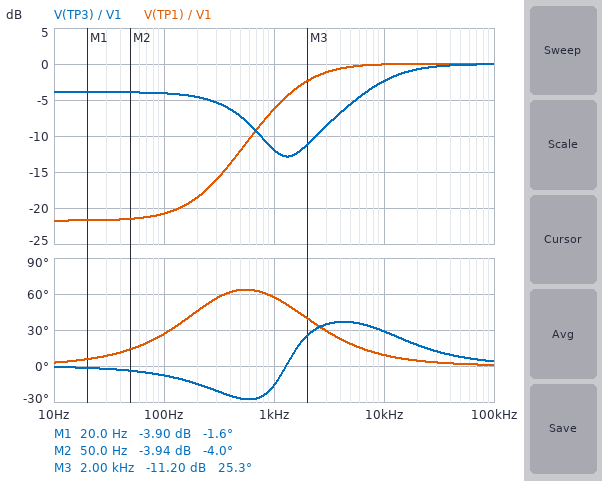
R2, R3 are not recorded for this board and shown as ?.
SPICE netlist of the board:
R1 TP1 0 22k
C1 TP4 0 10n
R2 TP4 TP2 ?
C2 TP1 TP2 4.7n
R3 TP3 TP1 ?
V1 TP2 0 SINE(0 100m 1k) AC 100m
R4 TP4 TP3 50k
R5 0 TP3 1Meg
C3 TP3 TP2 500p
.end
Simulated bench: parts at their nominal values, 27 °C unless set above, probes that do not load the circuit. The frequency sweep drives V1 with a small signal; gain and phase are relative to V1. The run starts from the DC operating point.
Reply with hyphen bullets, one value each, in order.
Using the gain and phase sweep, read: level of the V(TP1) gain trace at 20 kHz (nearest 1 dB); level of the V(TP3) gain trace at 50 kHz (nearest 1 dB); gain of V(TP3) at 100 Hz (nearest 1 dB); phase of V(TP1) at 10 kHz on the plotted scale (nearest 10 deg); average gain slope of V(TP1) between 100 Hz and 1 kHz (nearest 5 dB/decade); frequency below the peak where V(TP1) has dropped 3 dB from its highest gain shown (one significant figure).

- 0 dB
- 0 dB
- -4 dB
- 10 deg
- 15 dB/decade
- 2 kHz
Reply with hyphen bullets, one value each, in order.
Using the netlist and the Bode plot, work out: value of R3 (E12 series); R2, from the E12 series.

- 150 kΩ
- 33 kΩ
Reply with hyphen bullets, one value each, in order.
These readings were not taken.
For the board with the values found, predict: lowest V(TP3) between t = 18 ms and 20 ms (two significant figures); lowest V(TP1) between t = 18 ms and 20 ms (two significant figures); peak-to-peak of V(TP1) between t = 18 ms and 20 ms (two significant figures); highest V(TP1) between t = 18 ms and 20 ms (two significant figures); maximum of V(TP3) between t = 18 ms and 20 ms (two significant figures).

- -25 mV
- -49 mV
- 97 mV
- 49 mV
- 25 mV
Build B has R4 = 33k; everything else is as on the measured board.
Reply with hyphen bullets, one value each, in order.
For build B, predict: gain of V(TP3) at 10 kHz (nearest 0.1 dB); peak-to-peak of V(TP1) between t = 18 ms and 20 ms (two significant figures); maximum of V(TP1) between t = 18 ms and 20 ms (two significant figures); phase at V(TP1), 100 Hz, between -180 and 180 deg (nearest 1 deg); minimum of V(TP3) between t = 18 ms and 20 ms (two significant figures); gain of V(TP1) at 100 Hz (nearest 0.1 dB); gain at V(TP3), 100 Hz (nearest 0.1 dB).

- -4.0 dB
- 96 mV
- 48 mV
- 24 deg
- -28 mV
- -20.3 dB
- -3.4 dB
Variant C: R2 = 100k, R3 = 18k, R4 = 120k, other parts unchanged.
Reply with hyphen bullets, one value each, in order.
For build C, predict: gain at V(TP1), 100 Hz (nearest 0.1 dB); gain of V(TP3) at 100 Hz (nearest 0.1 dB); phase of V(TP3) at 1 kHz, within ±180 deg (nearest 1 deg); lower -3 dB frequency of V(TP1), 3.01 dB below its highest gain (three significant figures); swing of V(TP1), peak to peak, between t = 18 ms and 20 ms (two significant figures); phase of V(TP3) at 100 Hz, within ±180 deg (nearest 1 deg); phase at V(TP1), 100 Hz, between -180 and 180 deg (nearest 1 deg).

- -21.9 dB
- -17.5 dB
- 56 deg
- 1.71 kHz
- 100 mV
- 3 deg
- 23 deg
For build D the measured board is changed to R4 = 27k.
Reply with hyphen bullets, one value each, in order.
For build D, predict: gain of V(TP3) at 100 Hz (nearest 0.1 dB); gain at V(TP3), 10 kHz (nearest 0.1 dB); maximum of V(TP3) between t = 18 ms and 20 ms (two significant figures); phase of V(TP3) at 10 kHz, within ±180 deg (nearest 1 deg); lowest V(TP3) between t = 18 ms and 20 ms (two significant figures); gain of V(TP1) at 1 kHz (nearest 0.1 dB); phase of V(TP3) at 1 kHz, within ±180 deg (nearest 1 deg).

- -3.1 dB
- -5.0 dB
- 30 mV
- 41 deg
- -30 mV
- -6.5 dB
- -35 deg
